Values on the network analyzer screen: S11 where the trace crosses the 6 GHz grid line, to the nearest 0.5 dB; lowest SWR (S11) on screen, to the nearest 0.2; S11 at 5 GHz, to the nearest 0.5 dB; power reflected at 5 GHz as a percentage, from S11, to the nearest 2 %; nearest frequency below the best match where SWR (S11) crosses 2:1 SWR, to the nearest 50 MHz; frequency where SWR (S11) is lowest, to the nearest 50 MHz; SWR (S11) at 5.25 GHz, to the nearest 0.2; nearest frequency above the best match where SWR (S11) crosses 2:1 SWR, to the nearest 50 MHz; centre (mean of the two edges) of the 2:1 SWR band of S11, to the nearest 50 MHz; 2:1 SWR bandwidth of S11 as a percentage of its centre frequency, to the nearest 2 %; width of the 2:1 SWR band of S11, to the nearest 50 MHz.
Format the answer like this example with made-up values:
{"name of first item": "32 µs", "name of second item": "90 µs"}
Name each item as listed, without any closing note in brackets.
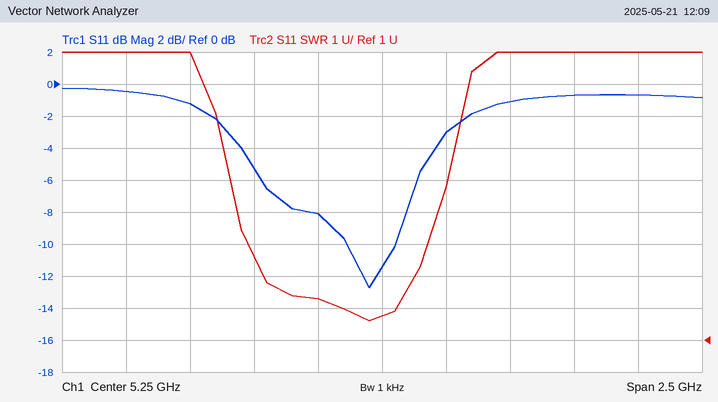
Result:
{"S11 where the trace crosses the 6 GHz grid line, to the nearest 0.5 dB": "-0.5 dB", "lowest SWR (S11) on screen, to the nearest 0.2": "1.6", "S11 at 5 GHz, to the nearest 0.5 dB": "-8.0 dB", "power reflected at 5 GHz as a percentage, from S11, to the nearest 2 %": "16 %", "nearest frequency below the best match where SWR (S11) crosses 2:1 SWR, to the nearest 50 MHz": "5.10 GHz", "frequency where SWR (S11) is lowest, to the nearest 50 MHz": "5.20 GHz", "SWR (S11) at 5.25 GHz, to the nearest 0.2": "1.8", "nearest frequency above the best match where SWR (S11) crosses 2:1 SWR, to the nearest 50 MHz": "5.30 GHz", "centre (mean of the two edges) of the 2:1 SWR band of S11, to the nearest 50 MHz": "5.20 GHz", "2:1 SWR bandwidth of S11 as a percentage of its centre frequency, to the nearest 2 %": "4 %", "width of the 2:1 SWR band of S11, to the nearest 50 MHz": "200 MHz"}
